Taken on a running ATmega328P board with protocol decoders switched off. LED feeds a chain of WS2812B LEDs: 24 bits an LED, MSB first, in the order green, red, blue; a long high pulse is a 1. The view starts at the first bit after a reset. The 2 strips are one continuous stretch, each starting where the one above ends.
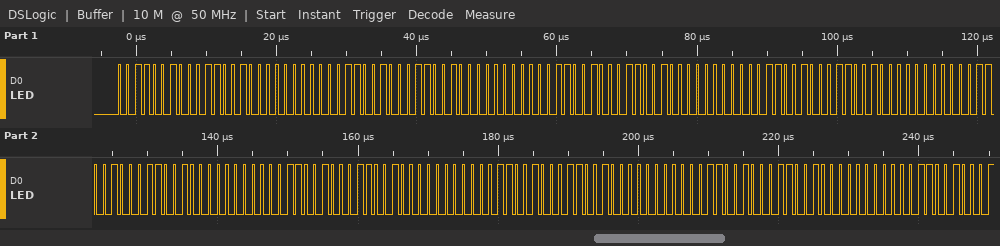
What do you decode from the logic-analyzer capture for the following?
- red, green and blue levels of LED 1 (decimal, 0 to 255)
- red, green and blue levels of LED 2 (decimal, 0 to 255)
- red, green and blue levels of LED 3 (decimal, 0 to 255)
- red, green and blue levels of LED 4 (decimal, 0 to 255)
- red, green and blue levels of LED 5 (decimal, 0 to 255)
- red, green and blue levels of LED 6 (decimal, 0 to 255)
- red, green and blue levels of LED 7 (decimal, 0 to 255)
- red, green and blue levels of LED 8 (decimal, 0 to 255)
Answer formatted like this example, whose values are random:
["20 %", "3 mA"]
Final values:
["50, 50, 0", "50, 50, 0", "50, 50, 0", "50, 50, 0", "50, 50, 0", "50, 50, 0", "50, 50, 0", "50, 50, 0"]
